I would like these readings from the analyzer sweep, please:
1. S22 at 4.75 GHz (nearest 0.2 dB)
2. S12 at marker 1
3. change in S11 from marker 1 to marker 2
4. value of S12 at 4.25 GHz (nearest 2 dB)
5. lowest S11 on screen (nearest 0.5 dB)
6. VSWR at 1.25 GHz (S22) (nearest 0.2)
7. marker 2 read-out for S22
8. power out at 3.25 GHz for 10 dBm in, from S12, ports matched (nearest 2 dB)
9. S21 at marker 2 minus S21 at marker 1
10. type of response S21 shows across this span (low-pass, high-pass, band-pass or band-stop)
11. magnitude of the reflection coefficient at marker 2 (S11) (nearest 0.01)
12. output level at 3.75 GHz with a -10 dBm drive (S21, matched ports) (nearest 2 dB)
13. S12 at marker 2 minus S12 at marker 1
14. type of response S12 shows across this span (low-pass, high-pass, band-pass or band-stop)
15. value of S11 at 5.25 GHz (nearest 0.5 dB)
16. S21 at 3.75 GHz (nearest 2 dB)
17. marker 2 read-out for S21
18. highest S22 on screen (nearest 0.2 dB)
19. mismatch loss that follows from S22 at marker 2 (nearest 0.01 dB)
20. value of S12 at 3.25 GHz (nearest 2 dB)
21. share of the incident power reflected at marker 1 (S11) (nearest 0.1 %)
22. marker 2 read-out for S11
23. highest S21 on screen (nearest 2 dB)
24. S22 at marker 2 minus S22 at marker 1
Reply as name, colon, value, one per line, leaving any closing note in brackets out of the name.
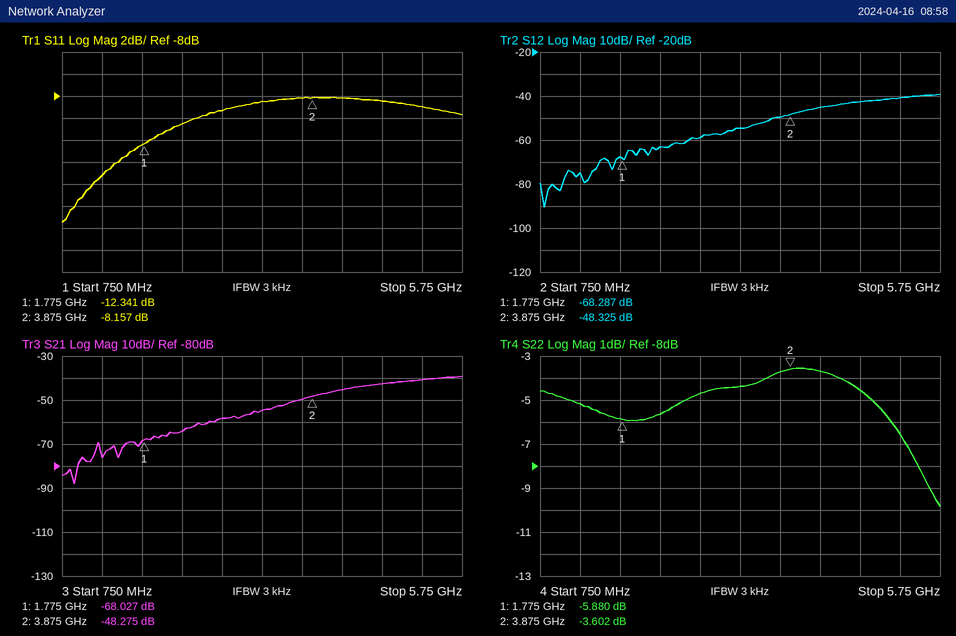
S22 at 4.75 GHz: -4.6 dB
S12 at marker 1: -68.287 dB
change in S11 from marker 1 to marker 2: 4.184 dB
value of S12 at 4.25 GHz: -46 dB
lowest S11 on screen: -19.5 dB
VSWR at 1.25 GHz (S22): 3.4
marker 2 read-out for S22: -3.602 dB
power out at 3.25 GHz for 10 dBm in, from S12, ports matched: -44 dBm
S21 at marker 2 minus S21 at marker 1: 19.752 dB
type of response S21 shows across this span: high-pass
magnitude of the reflection coefficient at marker 2 (S11): 0.39
output level at 3.75 GHz with a -10 dBm drive (S21, matched ports): -60 dBm
S12 at marker 2 minus S12 at marker 1: 19.962 dB
type of response S12 shows across this span: high-pass
value of S11 at 5.25 GHz: -9.0 dB
S21 at 3.75 GHz: -50 dB
marker 2 read-out for S21: -48.275 dB
highest S22 on screen: -3.6 dB
mismatch loss that follows from S22 at marker 2: 2.49 dB
value of S12 at 3.25 GHz: -54 dB
share of the incident power reflected at marker 1 (S11): 5.8 %
marker 2 read-out for S11: -8.157 dB
highest S21 on screen: -40 dB
S22 at marker 2 minus S22 at marker 1: 2.278 dB
